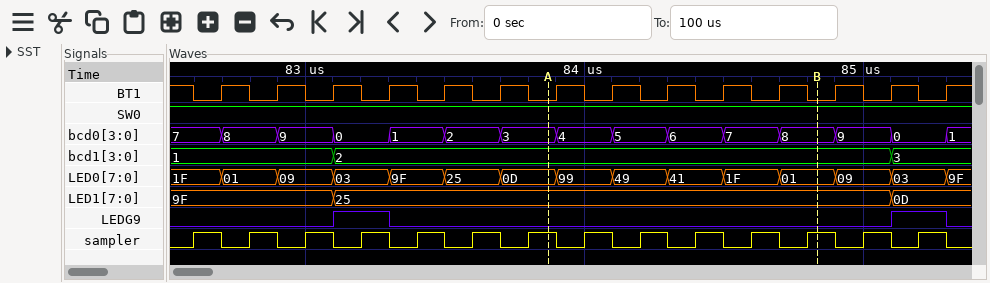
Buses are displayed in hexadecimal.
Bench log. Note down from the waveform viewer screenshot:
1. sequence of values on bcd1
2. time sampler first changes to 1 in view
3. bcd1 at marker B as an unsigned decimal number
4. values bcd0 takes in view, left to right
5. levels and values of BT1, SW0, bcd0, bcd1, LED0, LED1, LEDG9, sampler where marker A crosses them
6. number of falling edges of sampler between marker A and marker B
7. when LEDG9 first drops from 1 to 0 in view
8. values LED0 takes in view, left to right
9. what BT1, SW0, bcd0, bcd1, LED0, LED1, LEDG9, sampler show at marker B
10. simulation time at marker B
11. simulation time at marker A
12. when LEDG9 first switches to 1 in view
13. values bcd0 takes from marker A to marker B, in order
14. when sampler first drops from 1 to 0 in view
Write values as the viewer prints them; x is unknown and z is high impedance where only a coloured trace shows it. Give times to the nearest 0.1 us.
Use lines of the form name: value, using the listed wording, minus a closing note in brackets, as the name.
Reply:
sequence of values on bcd1: 1, 2, 3
time sampler first changes to 1 in view: 82.6 us
bcd1 at marker B as an unsigned decimal number: 2
values bcd0 takes in view, left to right: 7, 8, 9, 0, 1, 2, 3, 4, 5, 6, 7, 8, 9, 0, 1
levels and values of BT1, SW0, bcd0, bcd1, LED0, LED1, LEDG9, sampler where marker A crosses them: BT1=0, SW0=1, bcd0=3, bcd1=2, LED0=0D, LED1=25, LEDG9=0, sampler=1
number of falling edges of sampler between marker A and marker B: 5
when LEDG9 first drops from 1 to 0 in view: 83.3 us
values LED0 takes in view, left to right: 1F, 01, 09, 03, 9F, 25, 0D, 99, 49, 41, 1F, 01, 09, 03, 9F
what BT1, SW0, bcd0, bcd1, LED0, LED1, LEDG9, sampler show at marker B: BT1=0, SW0=1, bcd0=8, bcd1=2, LED0=01, LED1=25, LEDG9=0, sampler=1
simulation time at marker B: 84.8 us
simulation time at marker A: 83.9 us
when LEDG9 first switches to 1 in view: 83.1 us
values bcd0 takes from marker A to marker B, in order: 3, 4, 5, 6, 7, 8
when sampler first drops from 1 to 0 in view: 82.7 us
